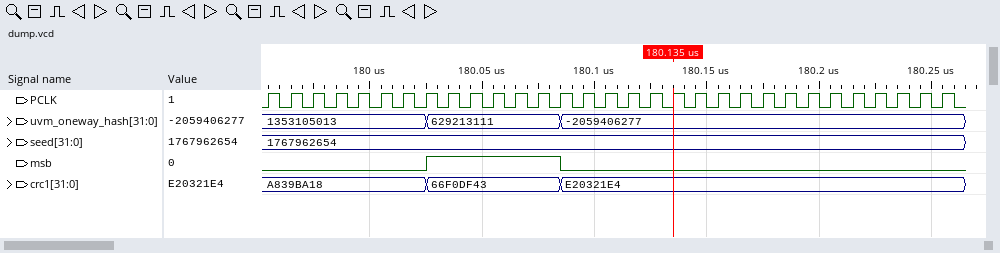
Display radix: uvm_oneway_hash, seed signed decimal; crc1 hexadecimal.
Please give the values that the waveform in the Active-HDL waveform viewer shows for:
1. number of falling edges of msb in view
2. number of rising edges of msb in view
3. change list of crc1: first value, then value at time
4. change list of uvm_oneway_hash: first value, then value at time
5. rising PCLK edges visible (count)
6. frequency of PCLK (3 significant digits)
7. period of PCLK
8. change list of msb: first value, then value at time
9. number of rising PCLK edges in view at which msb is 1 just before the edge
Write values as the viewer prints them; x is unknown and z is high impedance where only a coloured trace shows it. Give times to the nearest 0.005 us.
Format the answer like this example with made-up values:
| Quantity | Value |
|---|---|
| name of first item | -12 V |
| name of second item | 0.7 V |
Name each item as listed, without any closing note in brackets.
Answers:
| Quantity | Value |
|---|---|
| number of falling edges of msb in view | 1 |
| number of rising edges of msb in view | 1 |
| change list of crc1: first value, then value at time | A839BA18, 66F0DF43 at 180.025 us, E20321E4 at 180.085 us |
| change list of uvm_oneway_hash: first value, then value at time | 1353105013, 629213111 at 180.025 us, -2059406277 at 180.085 us |
| rising PCLK edges visible | 31 |
| frequency of PCLK | 100 MHz |
| period of PCLK | 0.01 us |
| change list of msb: first value, then value at time | 0, 1 at 180.025 us, 0 at 180.085 us |
| number of rising PCLK edges in view at which msb is 1 just before the edge | 6 |
